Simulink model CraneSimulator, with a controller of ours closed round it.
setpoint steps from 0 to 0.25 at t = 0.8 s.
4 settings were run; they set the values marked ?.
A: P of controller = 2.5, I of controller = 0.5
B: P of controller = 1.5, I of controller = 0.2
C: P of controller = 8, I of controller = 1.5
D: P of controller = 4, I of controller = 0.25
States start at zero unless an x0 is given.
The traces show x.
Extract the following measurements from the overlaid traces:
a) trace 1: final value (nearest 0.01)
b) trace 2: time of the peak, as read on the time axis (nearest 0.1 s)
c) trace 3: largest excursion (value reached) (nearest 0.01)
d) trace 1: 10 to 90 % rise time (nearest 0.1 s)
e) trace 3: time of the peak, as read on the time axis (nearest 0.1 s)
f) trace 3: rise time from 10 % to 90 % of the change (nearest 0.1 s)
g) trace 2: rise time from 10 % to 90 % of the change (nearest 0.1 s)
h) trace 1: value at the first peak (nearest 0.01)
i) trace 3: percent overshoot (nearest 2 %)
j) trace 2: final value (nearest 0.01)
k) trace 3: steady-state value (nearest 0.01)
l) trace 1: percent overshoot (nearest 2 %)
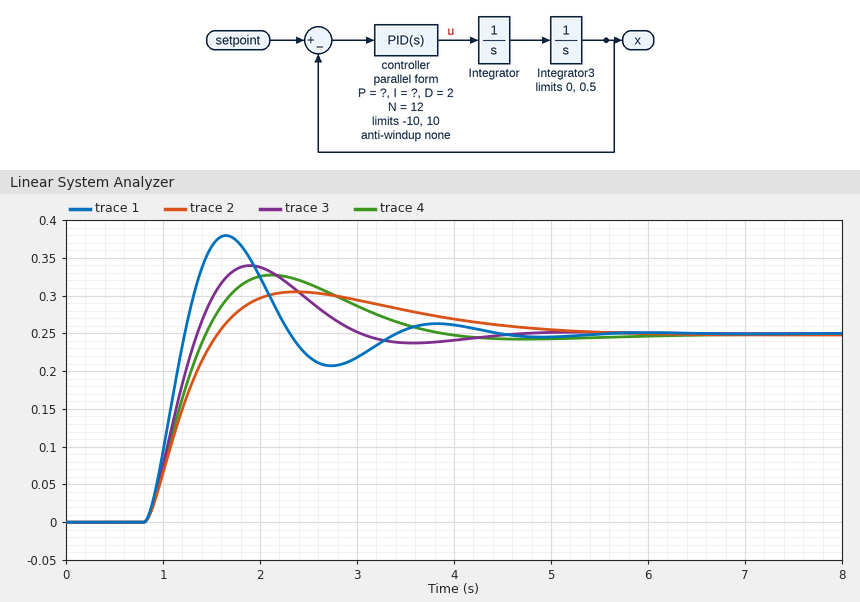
0.25
2.4 s
0.34
0.3 s
1.9 s
0.4 s
0.5 s
0.38
36 %
0.25
0.25
52 %
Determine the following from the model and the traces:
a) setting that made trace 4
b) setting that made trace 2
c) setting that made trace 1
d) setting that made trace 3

A
B
C
D
